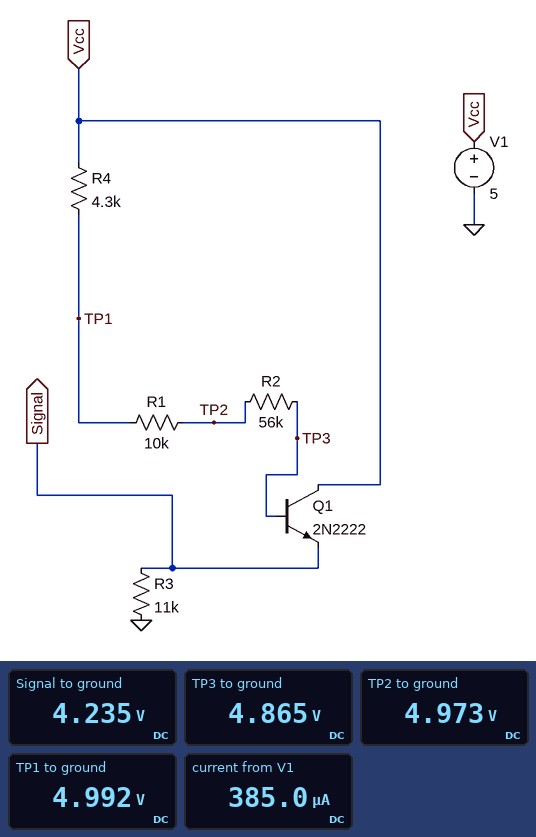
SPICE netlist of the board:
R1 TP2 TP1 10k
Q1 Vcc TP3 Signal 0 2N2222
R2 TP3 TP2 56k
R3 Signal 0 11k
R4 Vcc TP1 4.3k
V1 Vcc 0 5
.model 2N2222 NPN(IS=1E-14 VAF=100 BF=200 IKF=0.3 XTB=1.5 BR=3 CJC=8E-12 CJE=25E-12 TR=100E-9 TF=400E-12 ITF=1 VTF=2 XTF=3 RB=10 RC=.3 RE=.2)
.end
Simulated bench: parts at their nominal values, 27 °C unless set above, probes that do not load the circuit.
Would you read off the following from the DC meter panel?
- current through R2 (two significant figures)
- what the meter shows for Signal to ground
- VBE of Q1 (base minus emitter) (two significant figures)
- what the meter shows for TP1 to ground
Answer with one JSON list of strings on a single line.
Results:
["1.9 µA", "4.235 V", "630 mV", "4.992 V"]
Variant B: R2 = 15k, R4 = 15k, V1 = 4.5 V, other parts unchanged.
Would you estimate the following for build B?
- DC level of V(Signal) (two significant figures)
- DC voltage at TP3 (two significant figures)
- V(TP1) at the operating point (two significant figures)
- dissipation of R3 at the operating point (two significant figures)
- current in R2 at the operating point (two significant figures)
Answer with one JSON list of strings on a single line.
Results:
["3.8 V", "4.4 V", "4.5 V", "1.3 mW", "1.7 µA"]
